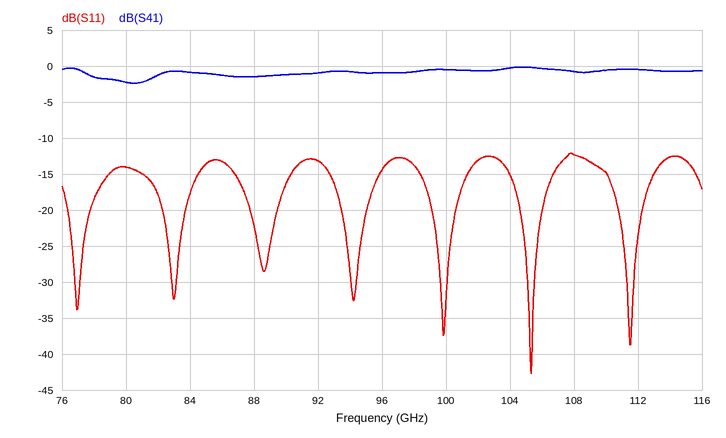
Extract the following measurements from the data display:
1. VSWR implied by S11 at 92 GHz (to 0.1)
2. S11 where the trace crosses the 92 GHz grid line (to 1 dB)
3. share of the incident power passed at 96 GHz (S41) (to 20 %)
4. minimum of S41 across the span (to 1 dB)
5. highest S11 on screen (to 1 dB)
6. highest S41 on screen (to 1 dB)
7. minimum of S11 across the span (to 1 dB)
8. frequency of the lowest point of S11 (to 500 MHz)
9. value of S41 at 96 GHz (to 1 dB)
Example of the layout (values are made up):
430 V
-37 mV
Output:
1.6
-13 dB
80 %
-2 dB
-12 dB
0 dB
-43 dB
105.5 GHz
-1 dB
